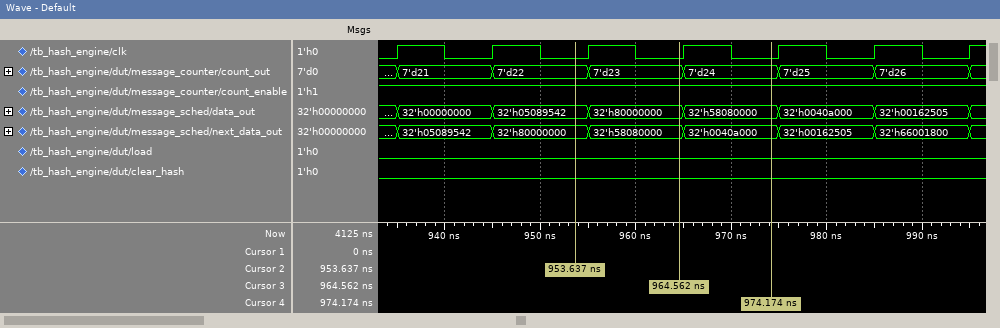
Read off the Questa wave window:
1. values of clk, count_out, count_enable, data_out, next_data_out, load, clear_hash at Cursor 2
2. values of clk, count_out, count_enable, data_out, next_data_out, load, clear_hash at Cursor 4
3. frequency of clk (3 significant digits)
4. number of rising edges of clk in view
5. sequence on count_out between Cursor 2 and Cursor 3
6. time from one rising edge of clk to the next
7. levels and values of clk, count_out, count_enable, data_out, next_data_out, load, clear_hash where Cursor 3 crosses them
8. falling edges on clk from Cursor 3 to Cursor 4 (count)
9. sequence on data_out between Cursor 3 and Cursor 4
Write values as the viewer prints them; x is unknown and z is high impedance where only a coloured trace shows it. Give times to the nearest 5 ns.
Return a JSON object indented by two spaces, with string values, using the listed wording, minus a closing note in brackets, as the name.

{
  "values of clk, count_out, count_enable, data_out, next_data_out, load, clear_hash at Cursor 2": "clk=0, count_out=7'd22, count_enable=1, data_out=32'h05089542, next_data_out=32'h80000000, load=0, clear_hash=0",
  "values of clk, count_out, count_enable, data_out, next_data_out, load, clear_hash at Cursor 4": "clk=0, count_out=7'd24, count_enable=1, data_out=32'h58080000, next_data_out=32'h0040a000, load=0, clear_hash=0",
  "frequency of clk": "100 MHz",
  "number of rising edges of clk in view": "7",
  "sequence on count_out between Cursor 2 and Cursor 3": "7'd22, 7'd23",
  "time from one rising edge of clk to the next": "10 ns",
  "levels and values of clk, count_out, count_enable, data_out, next_data_out, load, clear_hash where Cursor 3 crosses them": "clk=0, count_out=7'd23, count_enable=1, data_out=32'h80000000, next_data_out=32'h58080000, load=0, clear_hash=0",
  "falling edges on clk from Cursor 3 to Cursor 4": "1",
  "sequence on data_out between Cursor 3 and Cursor 4": "32'h80000000, 32'h58080000"
}
